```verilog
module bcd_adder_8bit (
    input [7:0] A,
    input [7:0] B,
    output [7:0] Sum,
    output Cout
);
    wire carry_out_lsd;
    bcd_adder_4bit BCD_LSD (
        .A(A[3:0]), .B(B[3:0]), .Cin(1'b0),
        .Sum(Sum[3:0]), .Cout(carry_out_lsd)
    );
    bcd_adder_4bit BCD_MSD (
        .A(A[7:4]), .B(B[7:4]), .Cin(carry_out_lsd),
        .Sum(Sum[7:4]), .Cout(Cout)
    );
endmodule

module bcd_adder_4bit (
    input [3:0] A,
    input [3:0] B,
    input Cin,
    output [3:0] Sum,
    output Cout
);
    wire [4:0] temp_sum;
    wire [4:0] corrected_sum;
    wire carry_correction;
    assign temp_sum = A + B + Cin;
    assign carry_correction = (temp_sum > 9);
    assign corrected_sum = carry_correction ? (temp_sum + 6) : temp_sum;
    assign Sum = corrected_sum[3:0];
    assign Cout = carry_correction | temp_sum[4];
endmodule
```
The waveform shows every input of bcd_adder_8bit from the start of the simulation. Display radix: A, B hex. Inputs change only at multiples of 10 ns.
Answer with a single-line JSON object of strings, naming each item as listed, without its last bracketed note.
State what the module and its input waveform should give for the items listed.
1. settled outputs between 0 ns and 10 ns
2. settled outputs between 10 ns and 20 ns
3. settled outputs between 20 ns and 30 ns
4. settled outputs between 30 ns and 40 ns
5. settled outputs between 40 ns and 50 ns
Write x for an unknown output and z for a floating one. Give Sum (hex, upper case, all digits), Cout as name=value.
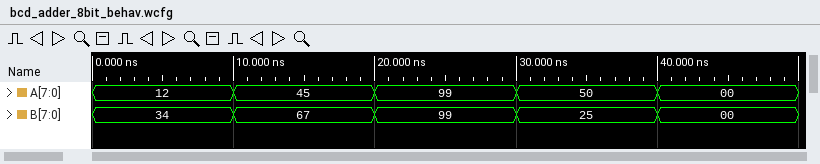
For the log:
{"settled outputs between 0 ns and 10 ns": "Sum=46, Cout=0", "settled outputs between 10 ns and 20 ns": "Sum=12, Cout=1", "settled outputs between 20 ns and 30 ns": "Sum=98, Cout=1", "settled outputs between 30 ns and 40 ns": "Sum=75, Cout=0", "settled outputs between 40 ns and 50 ns": "Sum=00, Cout=0"}
